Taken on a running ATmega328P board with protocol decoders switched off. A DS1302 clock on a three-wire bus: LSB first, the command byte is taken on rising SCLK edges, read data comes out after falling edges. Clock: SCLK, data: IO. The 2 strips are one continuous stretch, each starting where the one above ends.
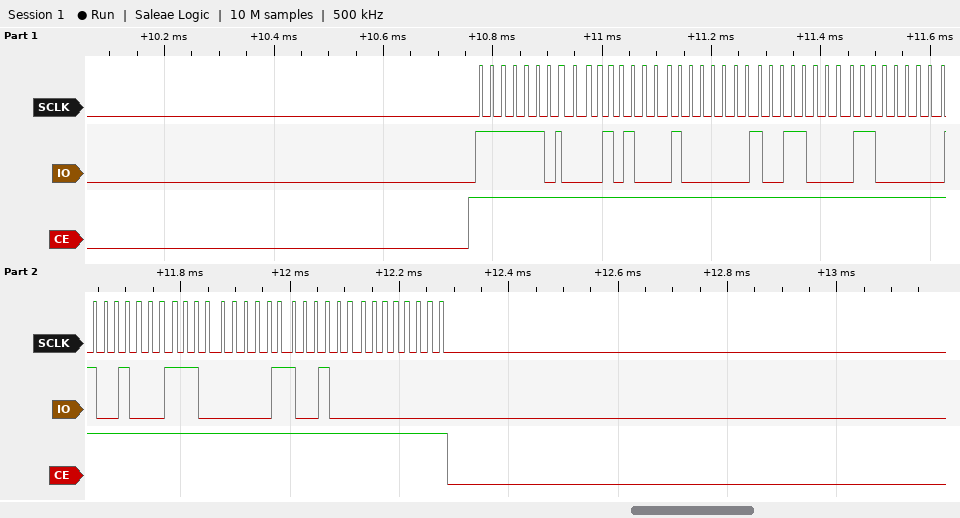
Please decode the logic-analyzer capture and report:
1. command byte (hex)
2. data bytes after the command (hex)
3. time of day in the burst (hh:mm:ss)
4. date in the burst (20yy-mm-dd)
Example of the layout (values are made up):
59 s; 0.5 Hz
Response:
0xBF; 28 02 19 06 12 07 26 00; 19:02:28; 2026-12-06
